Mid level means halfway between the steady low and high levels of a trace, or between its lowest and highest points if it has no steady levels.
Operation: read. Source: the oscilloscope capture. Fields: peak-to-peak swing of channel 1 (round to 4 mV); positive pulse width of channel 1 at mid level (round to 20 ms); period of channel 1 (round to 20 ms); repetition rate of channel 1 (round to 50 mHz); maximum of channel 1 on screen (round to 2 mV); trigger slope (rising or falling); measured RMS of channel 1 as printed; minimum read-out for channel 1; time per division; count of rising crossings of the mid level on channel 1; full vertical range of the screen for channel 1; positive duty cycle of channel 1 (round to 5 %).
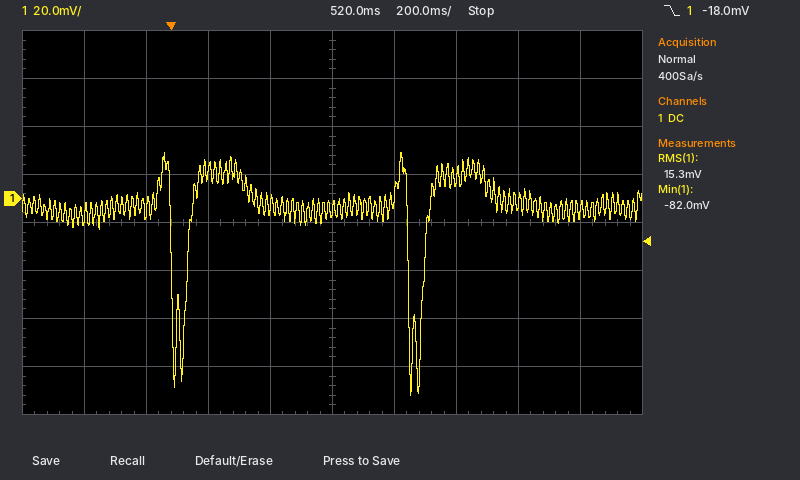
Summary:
100 mV
720 ms
760 ms
1.30 Hz
20 mV
falling
15.3 mV
-82.0 mV
200 ms
2
160 mV
95 %
